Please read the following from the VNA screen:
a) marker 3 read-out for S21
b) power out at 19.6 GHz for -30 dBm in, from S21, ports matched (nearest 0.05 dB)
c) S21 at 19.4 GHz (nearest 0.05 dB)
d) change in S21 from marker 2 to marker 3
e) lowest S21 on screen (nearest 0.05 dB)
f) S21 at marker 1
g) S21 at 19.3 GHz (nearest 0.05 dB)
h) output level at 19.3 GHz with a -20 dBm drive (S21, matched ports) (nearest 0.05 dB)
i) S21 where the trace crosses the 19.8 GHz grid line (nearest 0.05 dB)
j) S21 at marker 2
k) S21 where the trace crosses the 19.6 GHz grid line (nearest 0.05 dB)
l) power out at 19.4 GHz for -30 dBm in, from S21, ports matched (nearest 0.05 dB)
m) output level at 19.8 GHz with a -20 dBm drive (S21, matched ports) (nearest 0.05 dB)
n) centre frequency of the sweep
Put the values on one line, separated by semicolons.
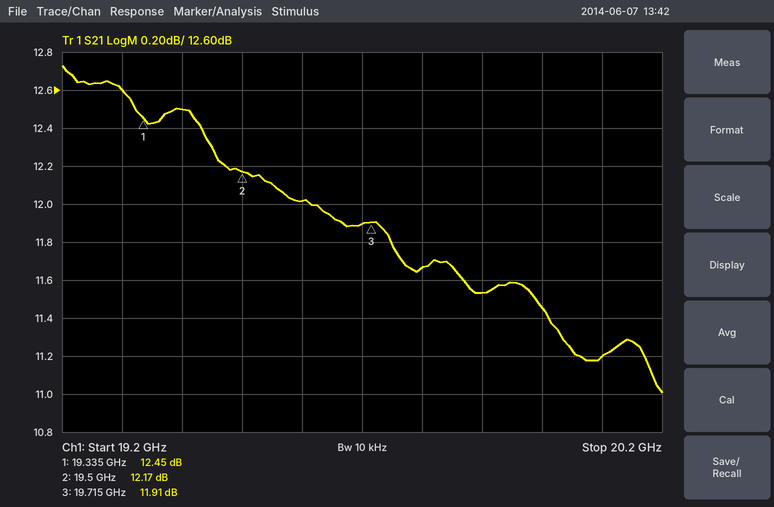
11.91 dB; -18.00 dBm; 12.50 dB; -0.26 dB; 11.00 dB; 12.45 dB; 12.60 dB; -7.40 dBm; 11.65 dB; 12.17 dB; 12.00 dB; -17.50 dBm; -8.35 dBm; 19.7 GHz
